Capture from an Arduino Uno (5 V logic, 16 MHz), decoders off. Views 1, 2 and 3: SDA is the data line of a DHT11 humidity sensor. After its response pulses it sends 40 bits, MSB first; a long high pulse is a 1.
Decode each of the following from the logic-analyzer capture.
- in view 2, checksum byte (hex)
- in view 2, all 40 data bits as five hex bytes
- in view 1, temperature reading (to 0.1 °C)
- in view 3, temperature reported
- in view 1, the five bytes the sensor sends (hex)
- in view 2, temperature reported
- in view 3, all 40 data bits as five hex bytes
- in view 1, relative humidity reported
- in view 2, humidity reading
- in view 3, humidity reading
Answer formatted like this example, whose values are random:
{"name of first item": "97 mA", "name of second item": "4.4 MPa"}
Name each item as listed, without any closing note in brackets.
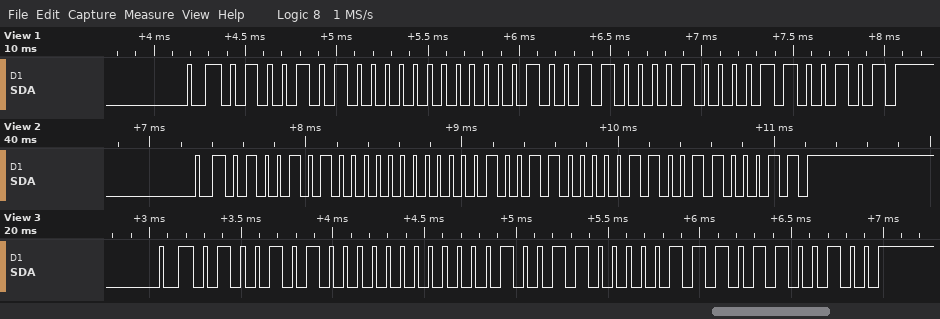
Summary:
{"in view 2, checksum byte": "0x63", "in view 2, all 40 data bits as five hex bytes": "4A 00 13 06 63", "in view 1, temperature reading": "19.8 °C", "in view 3, temperature reported": "19.7 °C", "in view 1, the five bytes the sensor sends": "4A 00 13 08 65", "in view 2, temperature reported": "19.6 °C", "in view 3, all 40 data bits as five hex bytes": "4A 00 13 07 64", "in view 1, relative humidity reported": "74 %", "in view 2, humidity reading": "74 %", "in view 3, humidity reading": "74 %"}
